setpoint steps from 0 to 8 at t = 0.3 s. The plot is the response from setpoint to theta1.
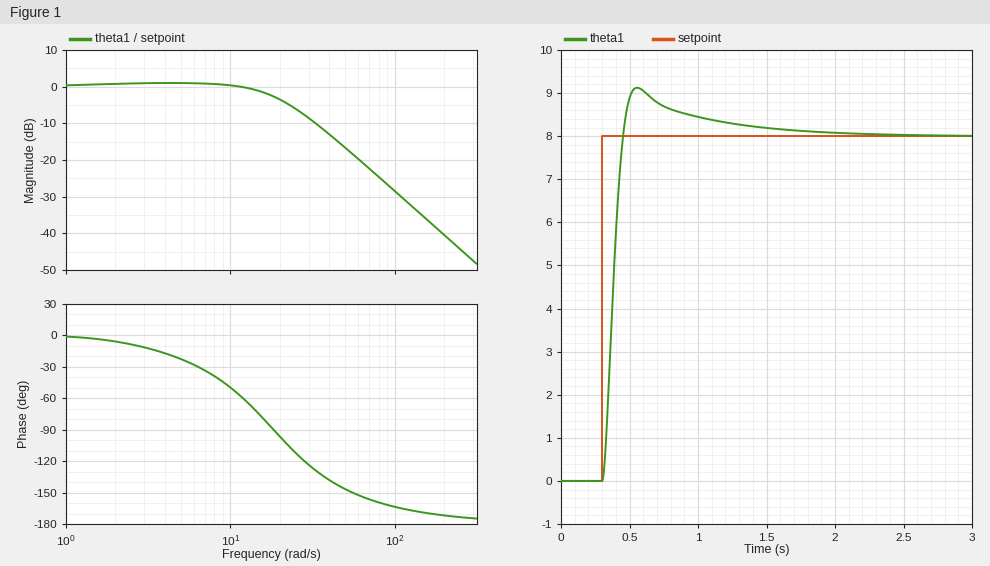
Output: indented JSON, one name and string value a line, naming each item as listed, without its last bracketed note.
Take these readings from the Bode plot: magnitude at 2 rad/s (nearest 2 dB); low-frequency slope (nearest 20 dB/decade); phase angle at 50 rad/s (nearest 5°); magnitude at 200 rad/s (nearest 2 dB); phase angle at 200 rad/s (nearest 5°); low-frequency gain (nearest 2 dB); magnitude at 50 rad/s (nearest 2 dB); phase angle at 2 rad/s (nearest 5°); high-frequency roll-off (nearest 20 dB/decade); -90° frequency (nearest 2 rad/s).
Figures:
{
  "magnitude at 2 rad/s": "0 dB",
  "low-frequency slope": "0 dB/decade",
  "phase angle at 50 rad/s": "-145°",
  "magnitude at 200 rad/s": "-40 dB",
  "phase angle at 200 rad/s": "-170°",
  "low-frequency gain": "0 dB",
  "magnitude at 50 rad/s": "-16 dB",
  "phase angle at 2 rad/s": "-5°",
  "high-frequency roll-off": "-40 dB/decade",
  "-90° frequency": "18 rad/s"
}
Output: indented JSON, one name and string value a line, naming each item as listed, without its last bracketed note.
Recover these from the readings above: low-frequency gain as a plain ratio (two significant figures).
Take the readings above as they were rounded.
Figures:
{
  "low-frequency gain as a plain ratio": "1.0"
}
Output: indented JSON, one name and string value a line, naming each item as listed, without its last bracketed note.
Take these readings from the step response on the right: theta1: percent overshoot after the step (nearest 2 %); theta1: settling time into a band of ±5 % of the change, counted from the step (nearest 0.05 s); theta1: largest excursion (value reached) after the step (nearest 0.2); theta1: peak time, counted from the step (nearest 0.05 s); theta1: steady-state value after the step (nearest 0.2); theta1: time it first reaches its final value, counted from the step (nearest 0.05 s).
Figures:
{
  "theta1: percent overshoot after the step": "14 %",
  "theta1: settling time into a band of ±5 % of the change, counted from the step": "0.75 s",
  "theta1: largest excursion (value reached) after the step": "9.2",
  "theta1: peak time, counted from the step": "0.25 s",
  "theta1: steady-state value after the step": "8.0",
  "theta1: time it first reaches its final value, counted from the step": "0.15 s"
}
